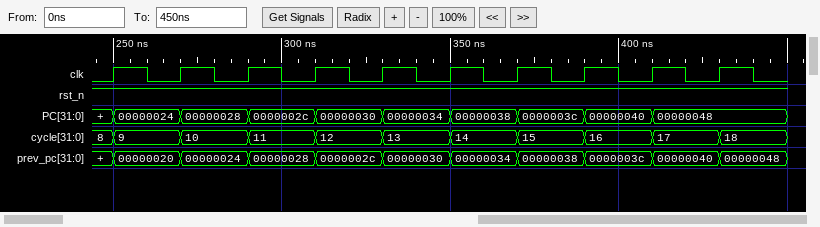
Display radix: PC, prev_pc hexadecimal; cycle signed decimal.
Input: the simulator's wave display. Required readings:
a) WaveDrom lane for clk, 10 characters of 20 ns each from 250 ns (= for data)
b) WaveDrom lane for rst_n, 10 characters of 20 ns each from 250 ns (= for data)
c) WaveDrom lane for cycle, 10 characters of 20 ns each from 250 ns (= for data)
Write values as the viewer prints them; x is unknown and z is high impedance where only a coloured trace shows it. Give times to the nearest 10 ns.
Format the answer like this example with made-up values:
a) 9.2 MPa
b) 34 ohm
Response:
a) {name: 'clk', wave: 'p.........'}
b) {name: 'rst_n', wave: '1.........'}
c) {name: 'cycle', wave: '==========', data: '9 10 11 12 13 14 15 16 17 18'}
